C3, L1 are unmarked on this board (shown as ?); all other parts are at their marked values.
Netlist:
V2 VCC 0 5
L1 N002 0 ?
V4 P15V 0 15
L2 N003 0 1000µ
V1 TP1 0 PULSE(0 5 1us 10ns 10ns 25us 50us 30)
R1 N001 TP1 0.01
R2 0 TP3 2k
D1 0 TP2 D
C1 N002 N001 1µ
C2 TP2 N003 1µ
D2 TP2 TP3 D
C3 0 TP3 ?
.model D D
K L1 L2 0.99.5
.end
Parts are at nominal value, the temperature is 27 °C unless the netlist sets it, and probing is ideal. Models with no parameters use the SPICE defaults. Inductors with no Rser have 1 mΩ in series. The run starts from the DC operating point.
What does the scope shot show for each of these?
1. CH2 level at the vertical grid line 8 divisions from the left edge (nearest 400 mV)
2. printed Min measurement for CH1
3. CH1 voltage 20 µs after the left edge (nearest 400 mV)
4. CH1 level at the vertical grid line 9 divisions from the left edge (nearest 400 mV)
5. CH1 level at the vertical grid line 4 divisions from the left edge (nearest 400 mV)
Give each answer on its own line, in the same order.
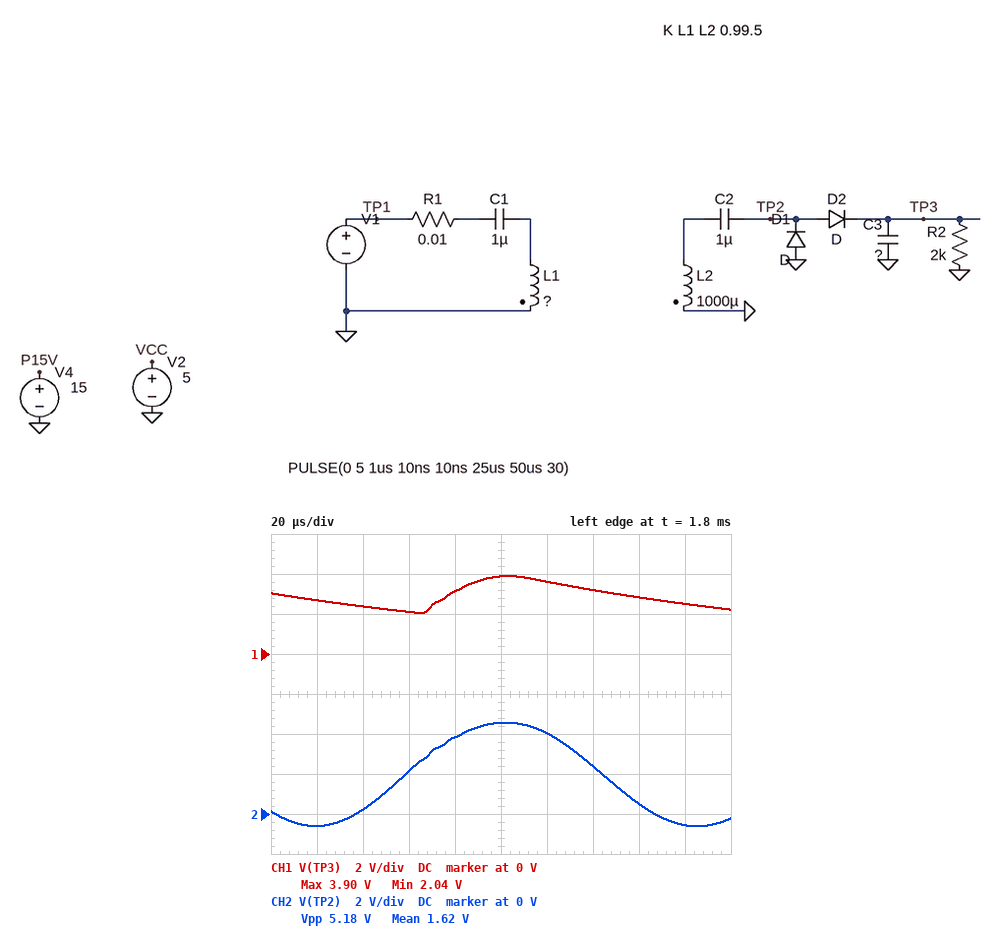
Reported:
400 mV
2.04 V
2.8 V
2.4 V
3.2 V
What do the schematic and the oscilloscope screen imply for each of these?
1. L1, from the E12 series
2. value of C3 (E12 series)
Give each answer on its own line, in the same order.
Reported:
680 µH
82 nF
